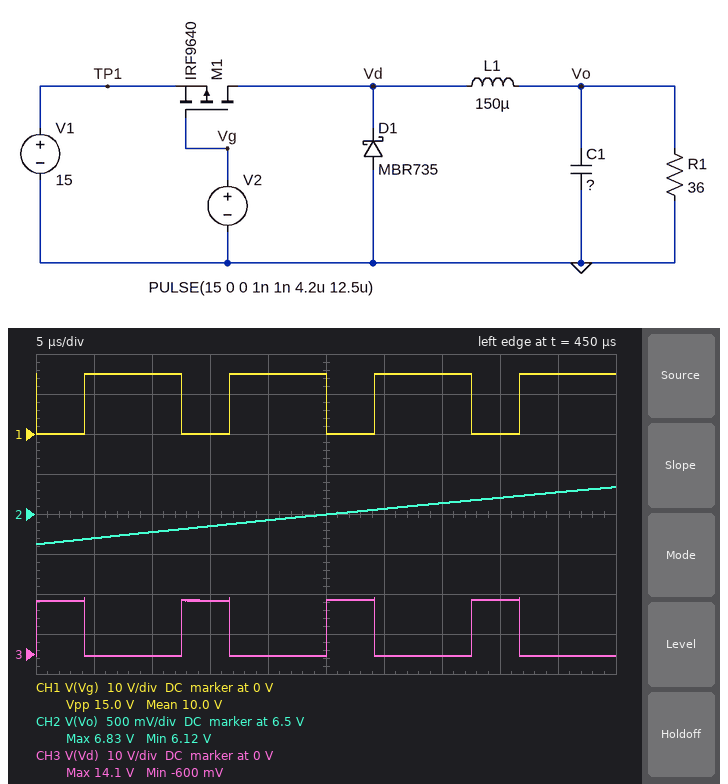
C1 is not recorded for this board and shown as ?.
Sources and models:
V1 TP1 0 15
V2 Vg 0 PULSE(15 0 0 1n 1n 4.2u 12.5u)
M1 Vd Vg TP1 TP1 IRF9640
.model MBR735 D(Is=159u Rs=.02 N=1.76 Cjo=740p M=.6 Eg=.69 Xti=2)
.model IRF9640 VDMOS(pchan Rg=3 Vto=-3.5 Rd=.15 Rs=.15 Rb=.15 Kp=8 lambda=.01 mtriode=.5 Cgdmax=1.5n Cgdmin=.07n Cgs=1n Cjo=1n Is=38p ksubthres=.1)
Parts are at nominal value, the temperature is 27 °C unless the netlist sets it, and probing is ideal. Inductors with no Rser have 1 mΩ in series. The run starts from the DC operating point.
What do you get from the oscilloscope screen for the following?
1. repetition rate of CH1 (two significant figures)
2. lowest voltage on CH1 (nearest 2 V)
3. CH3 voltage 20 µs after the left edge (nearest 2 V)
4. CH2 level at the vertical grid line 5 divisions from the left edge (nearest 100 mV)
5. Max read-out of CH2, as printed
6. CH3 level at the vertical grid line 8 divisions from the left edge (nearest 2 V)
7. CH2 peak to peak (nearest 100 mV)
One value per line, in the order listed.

80 kHz
0 V
0 V
6.5 V
6.83 V
14 V
700 mV
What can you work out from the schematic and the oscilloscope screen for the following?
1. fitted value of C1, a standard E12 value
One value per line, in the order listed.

330 µF
